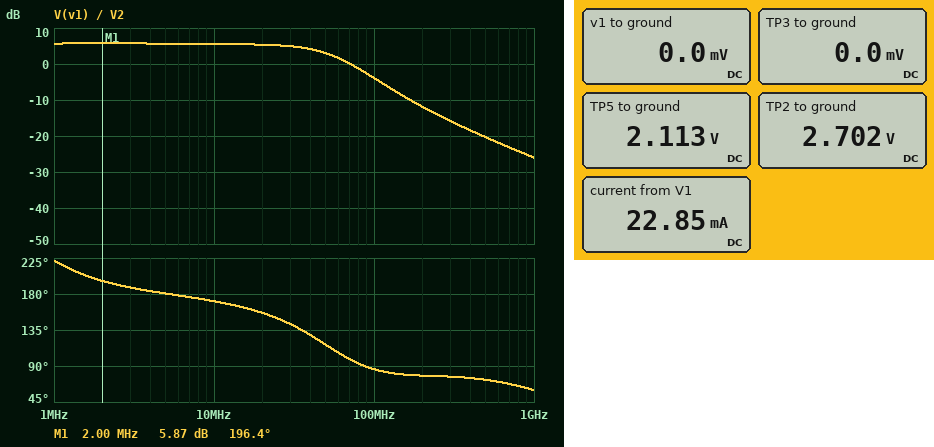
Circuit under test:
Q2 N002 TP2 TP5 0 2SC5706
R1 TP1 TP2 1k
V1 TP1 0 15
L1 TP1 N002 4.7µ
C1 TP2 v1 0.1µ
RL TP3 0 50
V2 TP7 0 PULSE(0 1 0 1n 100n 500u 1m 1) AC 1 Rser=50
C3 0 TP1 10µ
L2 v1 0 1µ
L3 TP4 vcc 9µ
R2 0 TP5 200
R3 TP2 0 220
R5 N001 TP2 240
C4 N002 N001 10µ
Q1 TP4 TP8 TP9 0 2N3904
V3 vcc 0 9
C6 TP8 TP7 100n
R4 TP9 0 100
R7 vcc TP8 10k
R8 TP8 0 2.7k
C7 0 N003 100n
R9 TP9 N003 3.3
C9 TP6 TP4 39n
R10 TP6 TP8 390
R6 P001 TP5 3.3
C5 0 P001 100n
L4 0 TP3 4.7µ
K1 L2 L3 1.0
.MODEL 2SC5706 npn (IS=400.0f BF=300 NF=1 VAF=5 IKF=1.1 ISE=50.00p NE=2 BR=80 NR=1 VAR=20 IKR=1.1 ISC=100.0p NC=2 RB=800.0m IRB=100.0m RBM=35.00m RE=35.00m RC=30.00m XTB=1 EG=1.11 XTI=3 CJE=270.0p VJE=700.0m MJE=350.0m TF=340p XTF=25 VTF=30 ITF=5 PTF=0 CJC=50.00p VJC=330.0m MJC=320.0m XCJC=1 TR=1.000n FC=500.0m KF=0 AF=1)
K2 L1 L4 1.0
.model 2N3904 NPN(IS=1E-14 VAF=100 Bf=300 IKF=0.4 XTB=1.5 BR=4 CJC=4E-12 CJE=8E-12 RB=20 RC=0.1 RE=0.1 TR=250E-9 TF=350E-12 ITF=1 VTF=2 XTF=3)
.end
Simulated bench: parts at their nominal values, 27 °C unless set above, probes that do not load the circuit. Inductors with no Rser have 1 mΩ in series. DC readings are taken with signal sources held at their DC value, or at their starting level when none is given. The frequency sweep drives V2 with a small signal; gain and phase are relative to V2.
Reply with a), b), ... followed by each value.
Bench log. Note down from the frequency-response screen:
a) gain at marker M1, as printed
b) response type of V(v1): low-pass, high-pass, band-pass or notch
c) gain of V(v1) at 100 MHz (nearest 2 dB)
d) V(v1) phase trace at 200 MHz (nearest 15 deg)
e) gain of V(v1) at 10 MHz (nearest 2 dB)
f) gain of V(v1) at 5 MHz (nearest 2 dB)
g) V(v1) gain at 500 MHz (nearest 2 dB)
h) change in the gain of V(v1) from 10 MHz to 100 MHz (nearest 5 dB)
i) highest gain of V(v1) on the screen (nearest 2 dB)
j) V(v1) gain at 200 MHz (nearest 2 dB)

a) 5.87 dB
b) low-pass
c) -4 dB
d) 75 deg
e) 6 dB
f) 6 dB
g) -20 dB
h) -10 dB
i) 6 dB
j) -12 dB
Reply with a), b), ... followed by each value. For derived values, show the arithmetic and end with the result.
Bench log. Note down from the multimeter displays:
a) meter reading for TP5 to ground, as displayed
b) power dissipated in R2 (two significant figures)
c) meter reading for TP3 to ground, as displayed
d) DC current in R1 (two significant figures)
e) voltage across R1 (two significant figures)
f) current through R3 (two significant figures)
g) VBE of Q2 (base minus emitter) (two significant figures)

a) 2.113 V
b) (2.113 V)^2 / 200 Ω = 22 mW
c) 0.0 mV
d) (15 V - 2.702 V) / 1 kΩ = 12 mA
e) 15 V - 2.702 V = 12 V
f) (2.702 V) / 220 Ω = 12 mA
g) 2.702 V - 2.113 V = 590 mV
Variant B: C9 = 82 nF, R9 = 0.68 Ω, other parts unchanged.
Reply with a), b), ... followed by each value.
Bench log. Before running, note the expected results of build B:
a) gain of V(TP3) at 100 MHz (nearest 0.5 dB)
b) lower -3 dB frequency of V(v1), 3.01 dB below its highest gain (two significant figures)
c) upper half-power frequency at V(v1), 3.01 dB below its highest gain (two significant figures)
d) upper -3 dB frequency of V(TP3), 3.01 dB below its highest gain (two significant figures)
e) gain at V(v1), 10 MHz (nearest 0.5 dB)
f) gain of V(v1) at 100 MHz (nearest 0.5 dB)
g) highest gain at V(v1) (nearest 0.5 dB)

a) 12.0 dB
b) 420 kHz
c) 49 MHz
d) 53 MHz
e) 6.5 dB
f) -3.0 dB
g) 8.0 dB
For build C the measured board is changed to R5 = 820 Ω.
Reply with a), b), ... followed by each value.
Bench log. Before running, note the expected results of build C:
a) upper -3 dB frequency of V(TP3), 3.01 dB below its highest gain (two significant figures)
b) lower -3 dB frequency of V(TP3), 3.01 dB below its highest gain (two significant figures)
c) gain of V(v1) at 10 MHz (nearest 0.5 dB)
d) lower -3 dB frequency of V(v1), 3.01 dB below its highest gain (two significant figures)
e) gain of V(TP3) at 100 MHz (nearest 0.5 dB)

a) 48 MHz
b) 1.7 MHz
c) 6.5 dB
d) 600 kHz
e) 12.0 dB
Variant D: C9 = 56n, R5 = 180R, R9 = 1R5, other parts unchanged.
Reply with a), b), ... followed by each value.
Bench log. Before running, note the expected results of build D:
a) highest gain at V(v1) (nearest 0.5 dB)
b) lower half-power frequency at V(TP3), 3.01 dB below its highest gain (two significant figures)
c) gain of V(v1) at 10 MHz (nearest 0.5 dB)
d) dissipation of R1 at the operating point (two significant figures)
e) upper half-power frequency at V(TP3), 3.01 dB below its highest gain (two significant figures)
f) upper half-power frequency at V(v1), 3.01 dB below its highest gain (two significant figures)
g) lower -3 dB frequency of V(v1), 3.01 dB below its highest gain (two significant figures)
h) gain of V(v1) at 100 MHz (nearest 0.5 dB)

a) 7.0 dB
b) 1.2 MHz
c) 6.0 dB
d) 150 mW
e) 52 MHz
f) 50 MHz
g) 440 kHz
h) -3.0 dB
